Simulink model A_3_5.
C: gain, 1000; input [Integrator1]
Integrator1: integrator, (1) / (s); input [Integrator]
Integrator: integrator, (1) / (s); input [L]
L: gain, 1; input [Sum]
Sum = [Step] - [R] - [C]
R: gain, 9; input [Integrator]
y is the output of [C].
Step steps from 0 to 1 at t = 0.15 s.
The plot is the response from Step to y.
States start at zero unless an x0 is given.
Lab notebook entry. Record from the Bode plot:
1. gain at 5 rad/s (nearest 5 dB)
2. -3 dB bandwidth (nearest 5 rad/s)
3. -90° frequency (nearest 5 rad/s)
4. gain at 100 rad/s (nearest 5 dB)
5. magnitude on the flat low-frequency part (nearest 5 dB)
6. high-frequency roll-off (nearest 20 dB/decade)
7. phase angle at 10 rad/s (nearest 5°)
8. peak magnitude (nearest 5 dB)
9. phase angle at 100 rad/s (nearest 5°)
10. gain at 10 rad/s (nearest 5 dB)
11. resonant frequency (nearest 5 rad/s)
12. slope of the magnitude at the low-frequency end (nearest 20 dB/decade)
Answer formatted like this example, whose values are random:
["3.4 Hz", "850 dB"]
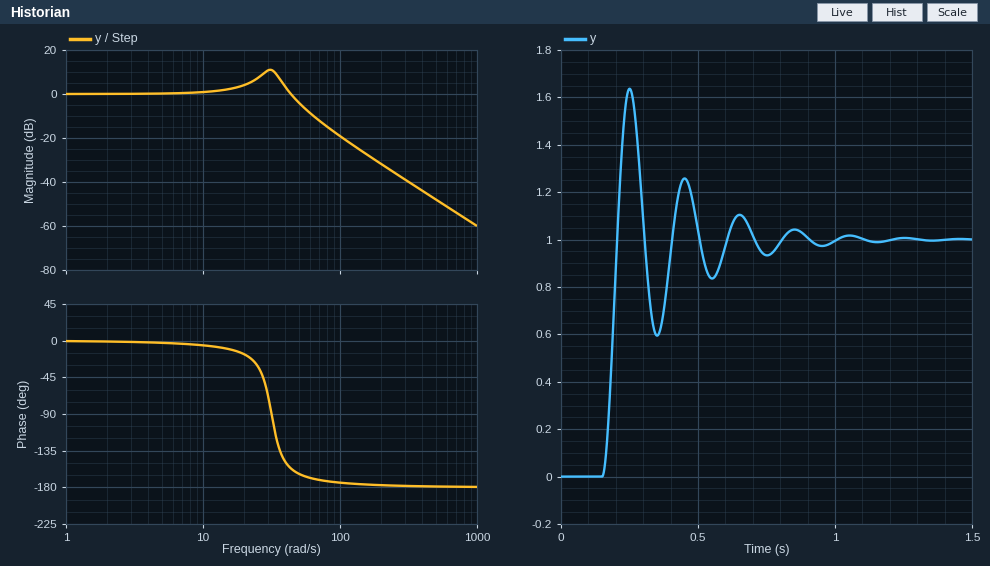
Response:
["0 dB", "50 rad/s", "30 rad/s", "-20 dB", "0 dB", "-40 dB/decade", "-5°", "10 dB", "-175°", "0 dB", "30 rad/s", "0 dB/decade"]
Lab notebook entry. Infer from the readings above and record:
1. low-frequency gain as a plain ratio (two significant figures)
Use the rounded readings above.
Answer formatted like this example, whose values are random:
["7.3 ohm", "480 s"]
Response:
["1.0"]
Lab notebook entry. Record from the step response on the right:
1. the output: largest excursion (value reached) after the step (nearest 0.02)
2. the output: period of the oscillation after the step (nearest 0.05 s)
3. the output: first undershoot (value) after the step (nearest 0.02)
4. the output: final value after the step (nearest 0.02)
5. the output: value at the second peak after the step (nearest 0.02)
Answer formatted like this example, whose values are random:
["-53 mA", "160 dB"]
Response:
["1.64", "0.20 s", "0.60", "1.00", "1.26"]
